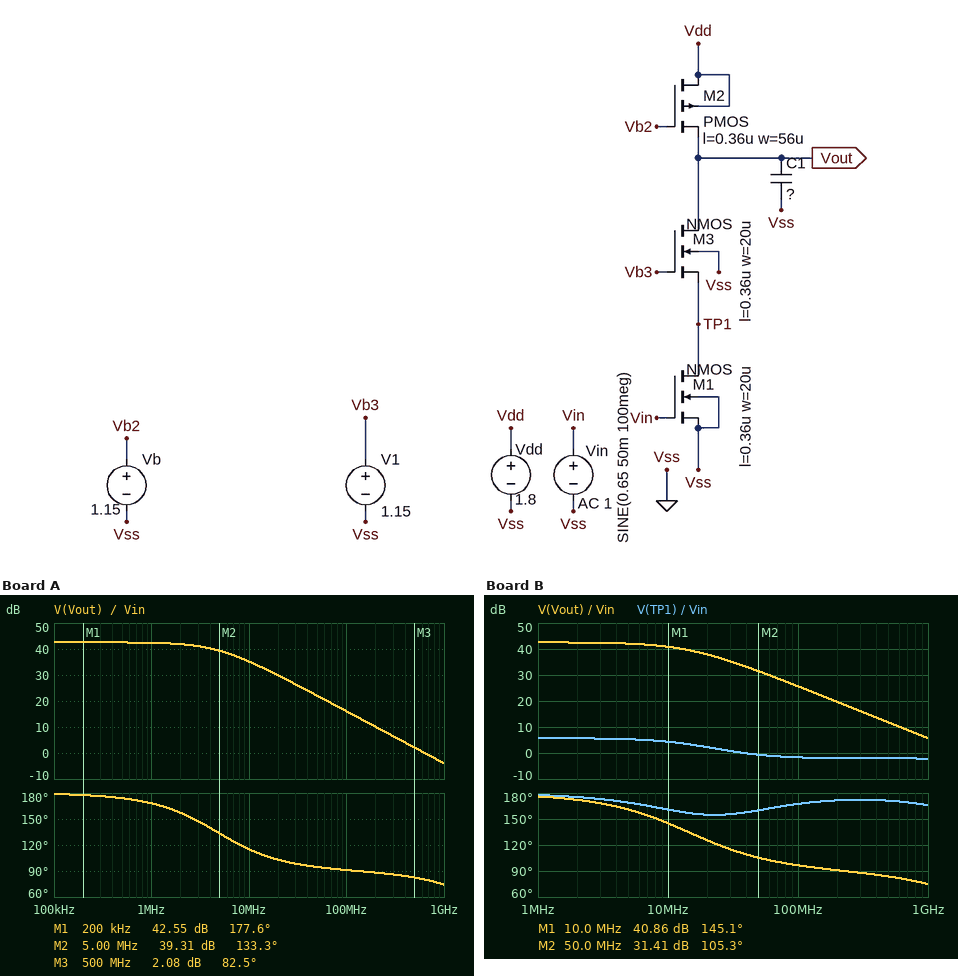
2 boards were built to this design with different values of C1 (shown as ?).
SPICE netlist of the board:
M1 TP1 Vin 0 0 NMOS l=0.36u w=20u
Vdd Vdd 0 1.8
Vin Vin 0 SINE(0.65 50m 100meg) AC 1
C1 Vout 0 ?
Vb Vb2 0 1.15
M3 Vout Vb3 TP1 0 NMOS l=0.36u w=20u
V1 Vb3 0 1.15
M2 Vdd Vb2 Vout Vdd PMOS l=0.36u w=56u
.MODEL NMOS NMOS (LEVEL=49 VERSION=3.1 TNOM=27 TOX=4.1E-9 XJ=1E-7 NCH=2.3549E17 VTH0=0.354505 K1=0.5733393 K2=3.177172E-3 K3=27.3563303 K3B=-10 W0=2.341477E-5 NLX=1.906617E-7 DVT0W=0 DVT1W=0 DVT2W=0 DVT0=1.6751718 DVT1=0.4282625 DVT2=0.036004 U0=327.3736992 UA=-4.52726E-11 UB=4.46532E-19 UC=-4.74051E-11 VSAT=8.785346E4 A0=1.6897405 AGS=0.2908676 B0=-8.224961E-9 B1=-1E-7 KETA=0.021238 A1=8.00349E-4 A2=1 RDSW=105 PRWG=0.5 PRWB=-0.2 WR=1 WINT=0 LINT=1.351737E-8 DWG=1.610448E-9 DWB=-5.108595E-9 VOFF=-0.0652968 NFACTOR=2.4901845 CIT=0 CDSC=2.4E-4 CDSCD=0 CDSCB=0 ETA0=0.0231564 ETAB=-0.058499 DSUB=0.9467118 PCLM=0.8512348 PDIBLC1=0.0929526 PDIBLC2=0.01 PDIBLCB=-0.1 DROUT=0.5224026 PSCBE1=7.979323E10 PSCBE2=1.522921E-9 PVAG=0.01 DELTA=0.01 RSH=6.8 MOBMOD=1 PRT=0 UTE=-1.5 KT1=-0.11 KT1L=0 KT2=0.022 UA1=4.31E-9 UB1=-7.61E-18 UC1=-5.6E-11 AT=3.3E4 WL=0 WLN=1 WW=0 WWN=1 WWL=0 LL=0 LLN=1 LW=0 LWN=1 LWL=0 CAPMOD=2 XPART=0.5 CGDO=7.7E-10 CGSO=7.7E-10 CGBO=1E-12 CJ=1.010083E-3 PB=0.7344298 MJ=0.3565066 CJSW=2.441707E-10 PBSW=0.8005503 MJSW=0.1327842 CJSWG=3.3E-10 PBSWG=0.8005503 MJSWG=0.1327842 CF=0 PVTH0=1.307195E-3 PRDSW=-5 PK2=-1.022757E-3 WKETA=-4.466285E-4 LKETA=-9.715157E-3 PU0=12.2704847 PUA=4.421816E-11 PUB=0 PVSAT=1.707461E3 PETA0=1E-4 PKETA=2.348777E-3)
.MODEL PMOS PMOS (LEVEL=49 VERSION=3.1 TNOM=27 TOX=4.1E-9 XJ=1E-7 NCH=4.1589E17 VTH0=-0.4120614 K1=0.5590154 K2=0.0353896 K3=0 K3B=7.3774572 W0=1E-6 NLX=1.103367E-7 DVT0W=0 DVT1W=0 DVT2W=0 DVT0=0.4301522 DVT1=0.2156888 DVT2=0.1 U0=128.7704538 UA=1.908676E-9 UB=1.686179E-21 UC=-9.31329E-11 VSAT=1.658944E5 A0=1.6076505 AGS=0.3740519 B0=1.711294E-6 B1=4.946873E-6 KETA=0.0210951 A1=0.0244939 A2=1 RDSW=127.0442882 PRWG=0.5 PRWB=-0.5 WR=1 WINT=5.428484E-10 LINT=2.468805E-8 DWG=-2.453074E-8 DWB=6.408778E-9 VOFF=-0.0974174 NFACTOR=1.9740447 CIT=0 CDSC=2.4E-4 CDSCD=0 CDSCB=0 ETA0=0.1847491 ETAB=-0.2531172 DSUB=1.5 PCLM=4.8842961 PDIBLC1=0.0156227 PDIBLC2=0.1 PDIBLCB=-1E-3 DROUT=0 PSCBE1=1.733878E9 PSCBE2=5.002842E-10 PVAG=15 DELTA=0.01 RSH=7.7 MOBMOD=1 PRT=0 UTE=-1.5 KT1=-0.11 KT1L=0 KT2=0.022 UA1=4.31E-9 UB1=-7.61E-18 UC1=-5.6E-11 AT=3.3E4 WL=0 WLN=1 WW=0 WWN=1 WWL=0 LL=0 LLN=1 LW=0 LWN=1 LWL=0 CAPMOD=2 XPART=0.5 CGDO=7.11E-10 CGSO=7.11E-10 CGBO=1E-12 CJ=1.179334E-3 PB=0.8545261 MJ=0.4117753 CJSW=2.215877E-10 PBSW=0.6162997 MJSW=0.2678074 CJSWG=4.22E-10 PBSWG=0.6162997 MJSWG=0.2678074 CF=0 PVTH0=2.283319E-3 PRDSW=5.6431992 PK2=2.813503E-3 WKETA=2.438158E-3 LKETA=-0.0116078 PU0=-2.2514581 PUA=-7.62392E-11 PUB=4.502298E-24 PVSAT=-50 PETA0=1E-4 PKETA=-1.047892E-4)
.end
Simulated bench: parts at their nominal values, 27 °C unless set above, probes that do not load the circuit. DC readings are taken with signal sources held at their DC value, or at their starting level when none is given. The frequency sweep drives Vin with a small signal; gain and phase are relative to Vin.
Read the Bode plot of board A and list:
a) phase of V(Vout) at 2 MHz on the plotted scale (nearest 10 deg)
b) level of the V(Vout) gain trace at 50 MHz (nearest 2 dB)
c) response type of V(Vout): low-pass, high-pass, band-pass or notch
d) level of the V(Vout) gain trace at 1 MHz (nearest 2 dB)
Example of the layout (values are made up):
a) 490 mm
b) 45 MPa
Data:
a) 160 deg
b) 22 dB
c) low-pass
d) 42 dB
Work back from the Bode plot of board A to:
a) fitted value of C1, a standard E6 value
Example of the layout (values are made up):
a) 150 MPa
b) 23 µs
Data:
a) 470 fF
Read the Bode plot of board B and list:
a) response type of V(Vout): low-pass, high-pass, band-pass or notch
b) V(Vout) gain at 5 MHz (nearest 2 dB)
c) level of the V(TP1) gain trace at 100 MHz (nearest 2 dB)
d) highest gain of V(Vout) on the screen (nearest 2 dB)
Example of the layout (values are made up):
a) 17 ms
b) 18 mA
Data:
a) low-pass
b) 42 dB
c) -2 dB
d) 42 dB
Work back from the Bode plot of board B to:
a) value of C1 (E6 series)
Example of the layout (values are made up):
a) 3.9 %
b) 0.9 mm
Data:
a) 100 fF
